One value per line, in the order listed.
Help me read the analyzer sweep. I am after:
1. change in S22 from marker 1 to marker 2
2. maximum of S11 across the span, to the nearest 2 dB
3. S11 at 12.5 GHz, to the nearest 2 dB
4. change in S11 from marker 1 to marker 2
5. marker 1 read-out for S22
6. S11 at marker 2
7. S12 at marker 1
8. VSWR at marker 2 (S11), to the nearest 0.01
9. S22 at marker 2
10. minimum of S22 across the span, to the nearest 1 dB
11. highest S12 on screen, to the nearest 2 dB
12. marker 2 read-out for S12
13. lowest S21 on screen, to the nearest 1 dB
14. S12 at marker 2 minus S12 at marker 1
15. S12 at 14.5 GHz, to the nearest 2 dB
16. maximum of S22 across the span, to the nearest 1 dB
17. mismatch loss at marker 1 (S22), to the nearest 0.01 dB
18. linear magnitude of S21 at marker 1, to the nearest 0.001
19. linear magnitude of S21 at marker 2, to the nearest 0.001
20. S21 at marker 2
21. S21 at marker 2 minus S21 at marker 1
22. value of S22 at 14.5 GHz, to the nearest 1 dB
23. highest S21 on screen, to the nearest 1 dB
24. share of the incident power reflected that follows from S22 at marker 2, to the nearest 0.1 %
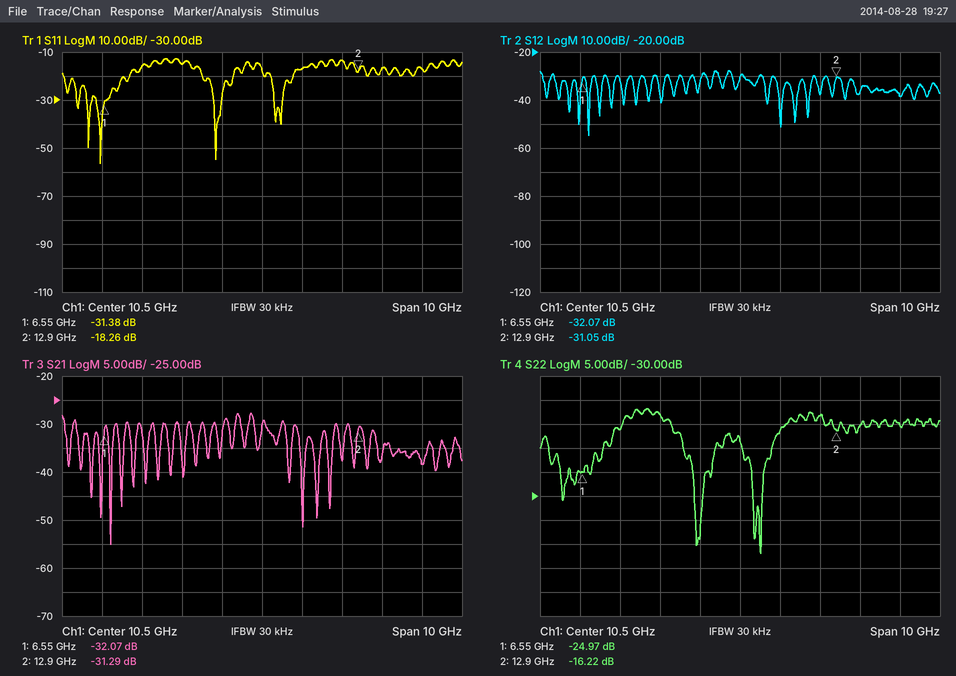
8.75 dB
-12 dB
-14 dB
13.12 dB
-24.97 dB
-18.26 dB
-32.07 dB
1.28
-16.22 dB
-42 dB
-28 dB
-31.05 dB
-55 dB
1.02 dB
-38 dB
-12 dB
0.01 dB
0.025
0.027
-31.29 dB
0.78 dB
-15 dB
-28 dB
2.4 %
